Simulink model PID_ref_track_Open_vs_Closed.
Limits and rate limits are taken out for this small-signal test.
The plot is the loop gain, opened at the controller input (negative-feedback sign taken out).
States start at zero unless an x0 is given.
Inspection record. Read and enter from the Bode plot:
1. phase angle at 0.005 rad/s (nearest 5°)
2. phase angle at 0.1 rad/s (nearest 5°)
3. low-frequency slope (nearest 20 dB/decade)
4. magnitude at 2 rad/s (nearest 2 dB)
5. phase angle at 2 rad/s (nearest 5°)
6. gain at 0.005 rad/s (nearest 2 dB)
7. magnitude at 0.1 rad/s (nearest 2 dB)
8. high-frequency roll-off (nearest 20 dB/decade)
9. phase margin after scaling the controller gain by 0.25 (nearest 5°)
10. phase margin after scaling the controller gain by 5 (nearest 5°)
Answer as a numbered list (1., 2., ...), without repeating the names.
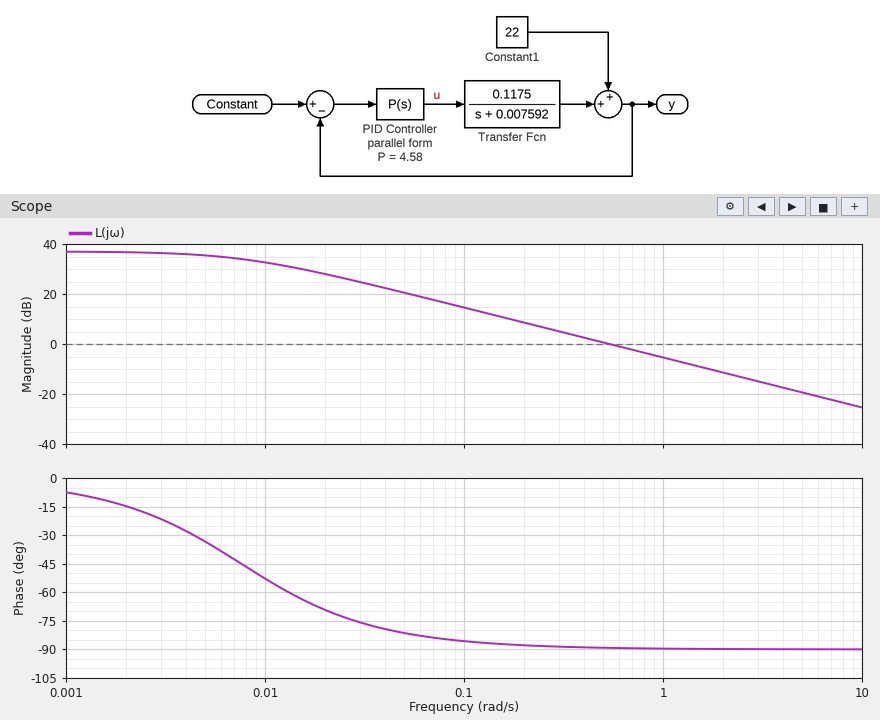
1. -35°
2. -85°
3. 0 dB/decade
4. -12 dB
5. -90°
6. 36 dB
7. 14 dB
8. -20 dB/decade
9. 95°
10. 90°
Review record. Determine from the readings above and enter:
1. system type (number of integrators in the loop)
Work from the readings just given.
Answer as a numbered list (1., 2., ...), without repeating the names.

1. 0
